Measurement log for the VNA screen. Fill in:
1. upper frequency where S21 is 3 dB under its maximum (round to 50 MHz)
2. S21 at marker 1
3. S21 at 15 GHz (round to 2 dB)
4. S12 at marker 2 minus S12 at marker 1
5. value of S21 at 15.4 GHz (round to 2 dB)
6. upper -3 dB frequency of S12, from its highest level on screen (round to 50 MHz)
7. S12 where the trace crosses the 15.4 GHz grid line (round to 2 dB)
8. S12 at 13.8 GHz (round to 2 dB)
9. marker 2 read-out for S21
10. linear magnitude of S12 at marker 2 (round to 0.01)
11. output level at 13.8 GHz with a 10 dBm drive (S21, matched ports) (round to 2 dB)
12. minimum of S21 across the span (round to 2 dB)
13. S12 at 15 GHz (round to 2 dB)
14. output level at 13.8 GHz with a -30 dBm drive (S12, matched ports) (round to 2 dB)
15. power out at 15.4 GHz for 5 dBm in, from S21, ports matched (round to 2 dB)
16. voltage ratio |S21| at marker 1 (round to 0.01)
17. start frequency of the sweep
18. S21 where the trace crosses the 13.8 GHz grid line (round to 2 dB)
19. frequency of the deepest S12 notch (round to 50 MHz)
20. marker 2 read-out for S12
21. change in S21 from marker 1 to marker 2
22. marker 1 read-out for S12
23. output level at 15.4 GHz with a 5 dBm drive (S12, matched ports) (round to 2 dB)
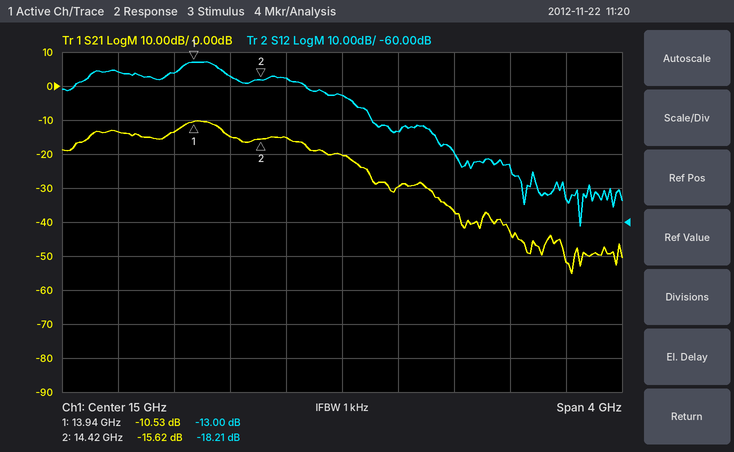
14.15 GHz
-10.53 dB
-20 dB
-5.21 dB
-30 dB
14.15 GHz
-34 dB
-16 dB
-15.62 dB
0.12
-4 dBm
-56 dB
-22 dB
-46 dBm
-24 dBm
0.30
13 GHz
-14 dB
16.70 GHz
-18.21 dB
-5.09 dB
-13.00 dB
-28 dBm
